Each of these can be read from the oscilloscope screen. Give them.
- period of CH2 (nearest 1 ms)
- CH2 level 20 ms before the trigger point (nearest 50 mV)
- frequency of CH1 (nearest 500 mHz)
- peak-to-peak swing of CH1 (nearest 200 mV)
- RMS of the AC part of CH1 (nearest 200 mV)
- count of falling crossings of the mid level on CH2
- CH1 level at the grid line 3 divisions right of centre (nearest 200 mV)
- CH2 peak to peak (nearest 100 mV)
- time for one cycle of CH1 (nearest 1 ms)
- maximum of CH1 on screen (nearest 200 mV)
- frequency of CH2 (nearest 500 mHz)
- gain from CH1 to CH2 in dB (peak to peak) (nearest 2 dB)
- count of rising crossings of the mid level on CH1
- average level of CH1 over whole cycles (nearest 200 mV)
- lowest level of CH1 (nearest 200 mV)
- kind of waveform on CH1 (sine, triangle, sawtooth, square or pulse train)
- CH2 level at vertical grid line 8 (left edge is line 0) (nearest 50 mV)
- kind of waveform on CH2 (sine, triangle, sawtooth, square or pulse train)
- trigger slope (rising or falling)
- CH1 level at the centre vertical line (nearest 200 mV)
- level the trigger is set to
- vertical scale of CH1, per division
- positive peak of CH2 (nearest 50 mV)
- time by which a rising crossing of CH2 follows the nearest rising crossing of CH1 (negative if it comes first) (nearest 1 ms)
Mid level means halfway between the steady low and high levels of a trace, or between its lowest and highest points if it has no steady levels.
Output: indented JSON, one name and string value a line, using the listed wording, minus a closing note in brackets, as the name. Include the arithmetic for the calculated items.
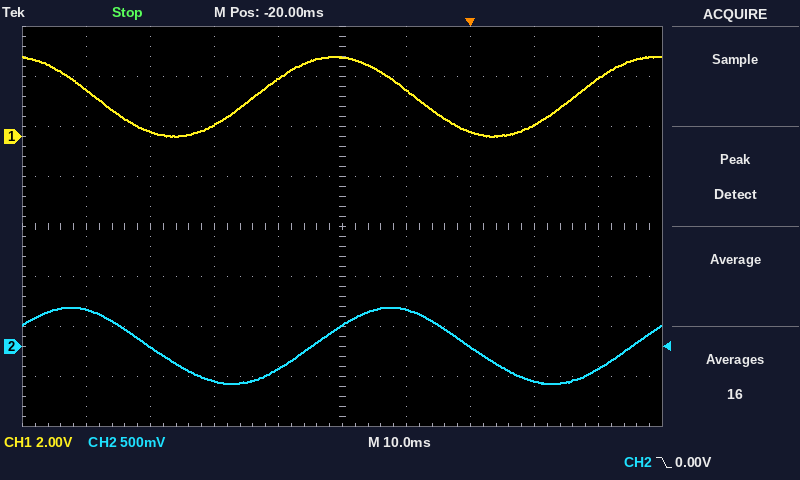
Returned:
{
  "period of CH2": "50 ms",
  "CH2 level 20 ms before the trigger point": "200 mV",
  "frequency of CH1": "1 / 50 ms ≈ 20.0 Hz",
  "peak-to-peak swing of CH1": "3.2 V − (0.0 V) = 3.2 V",
  "RMS of the AC part of CH1": "3.2 V / (2√2) ≈ 1.13 V, so 1.2 V to the nearest 200 mV",
  "count of falling crossings of the mid level on CH2": "2",
  "CH1 level at the grid line 3 divisions right of centre": "400 mV",
  "CH2 peak to peak": "800 mV",
  "time for one cycle of CH1": "50 ms",
  "maximum of CH1 on screen": "3.2 V",
  "frequency of CH2": "1 / 50 ms ≈ 20.0 Hz",
  "gain from CH1 to CH2 in dB (peak to peak)": "20 log10(800 mV / 3.2 V) ≈ -12 dB",
  "count of rising crossings of the mid level on CH1": "2",
  "average level of CH1 over whole cycles": "(3.2 V + (0.0 V)) / 2 ≈ 1.6 V",
  "lowest level of CH1": "0.0 V",
  "kind of waveform on CH1": "sine",
  "CH2 level at vertical grid line 8 (left edge is line 0)": "-350 mV",
  "kind of waveform on CH2": "sine",
  "trigger slope": "falling",
  "CH1 level at the centre vertical line": "3.2 V",
  "level the trigger is set to": "0.00 V",
  "vertical scale of CH1, per division": "2 V",
  "positive peak of CH2": "400 mV",
  "time by which a rising crossing of CH2 follows the nearest rising crossing of CH1 (negative if it comes first)": "+9 ms"
}
